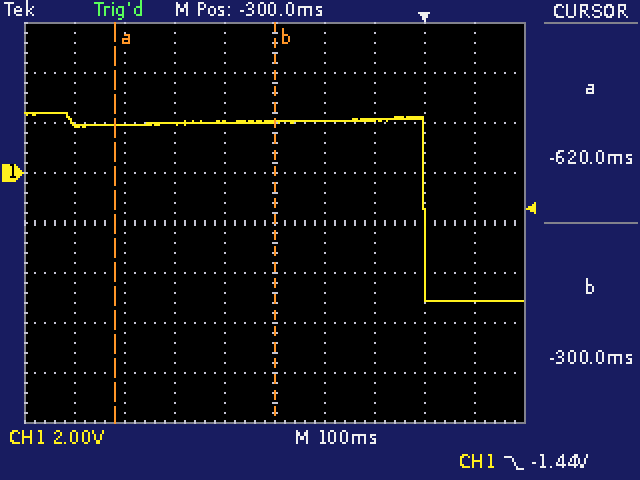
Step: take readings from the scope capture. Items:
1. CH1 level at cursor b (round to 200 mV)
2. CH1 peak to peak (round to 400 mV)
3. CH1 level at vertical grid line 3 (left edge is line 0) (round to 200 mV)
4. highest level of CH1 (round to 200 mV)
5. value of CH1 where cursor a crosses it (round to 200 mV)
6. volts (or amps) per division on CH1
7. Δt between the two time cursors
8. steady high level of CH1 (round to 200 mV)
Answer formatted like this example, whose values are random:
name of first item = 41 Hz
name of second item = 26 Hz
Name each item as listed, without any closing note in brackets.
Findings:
CH1 level at cursor b = 2.0 V
CH1 peak to peak = 7.6 V
CH1 level at vertical grid line 3 (left edge is line 0) = 2.0 V
highest level of CH1 = 2.4 V
value of CH1 where cursor a crosses it = 2.0 V
volts (or amps) per division on CH1 = 2 V
Δt between the two time cursors = 320 ms
steady high level of CH1 = 2.0 V
